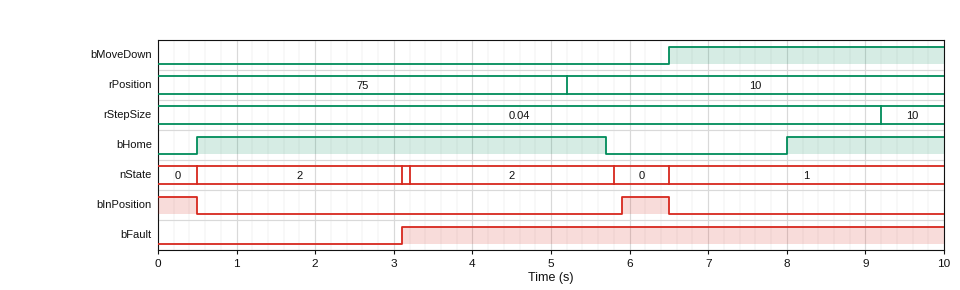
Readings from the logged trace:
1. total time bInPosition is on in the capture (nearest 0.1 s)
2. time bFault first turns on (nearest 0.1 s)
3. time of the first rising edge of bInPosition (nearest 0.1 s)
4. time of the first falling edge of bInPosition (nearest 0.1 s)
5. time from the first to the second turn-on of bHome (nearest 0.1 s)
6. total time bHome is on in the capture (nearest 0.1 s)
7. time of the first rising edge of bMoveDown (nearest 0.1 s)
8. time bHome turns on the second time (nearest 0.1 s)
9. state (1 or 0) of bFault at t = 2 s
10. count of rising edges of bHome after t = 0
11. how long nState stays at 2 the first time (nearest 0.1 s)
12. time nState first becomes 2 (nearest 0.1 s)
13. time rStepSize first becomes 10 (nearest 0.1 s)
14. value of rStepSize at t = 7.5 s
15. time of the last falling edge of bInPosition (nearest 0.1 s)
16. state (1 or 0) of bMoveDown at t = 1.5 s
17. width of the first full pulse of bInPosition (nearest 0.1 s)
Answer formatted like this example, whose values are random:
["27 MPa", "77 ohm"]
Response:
["1.1 s", "3.1 s", "5.9 s", "0.5 s", "7.5 s", "7.2 s", "6.5 s", "8.0 s", "0", "2", "2.6 s", "0.5 s", "9.2 s", "0.04", "6.5 s", "0", "0.6 s"]
